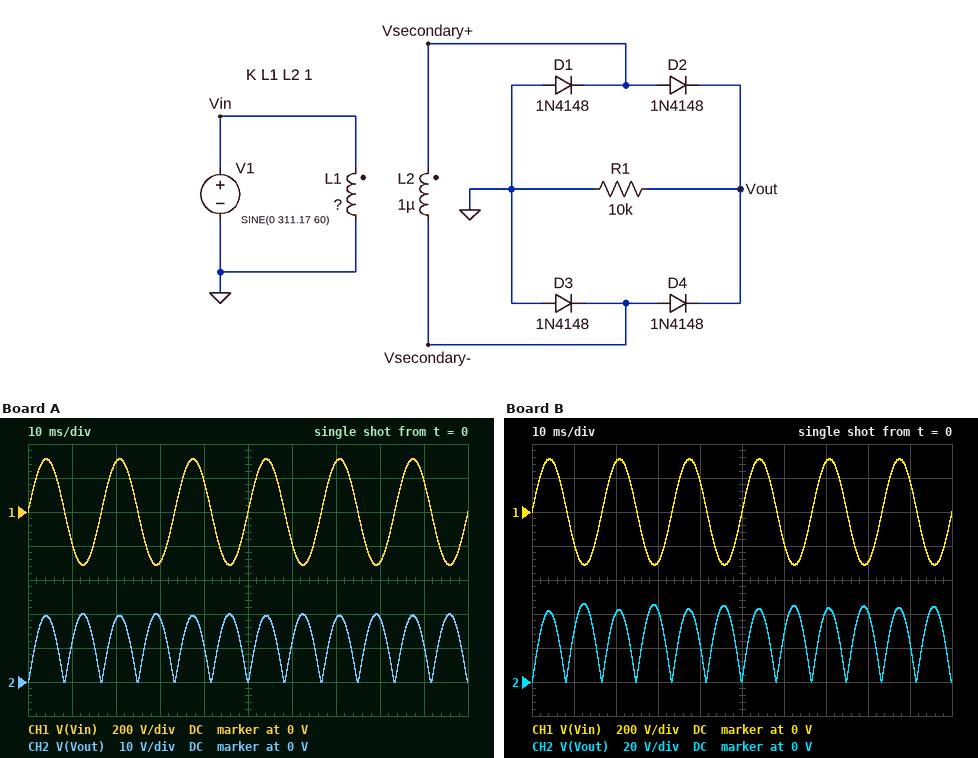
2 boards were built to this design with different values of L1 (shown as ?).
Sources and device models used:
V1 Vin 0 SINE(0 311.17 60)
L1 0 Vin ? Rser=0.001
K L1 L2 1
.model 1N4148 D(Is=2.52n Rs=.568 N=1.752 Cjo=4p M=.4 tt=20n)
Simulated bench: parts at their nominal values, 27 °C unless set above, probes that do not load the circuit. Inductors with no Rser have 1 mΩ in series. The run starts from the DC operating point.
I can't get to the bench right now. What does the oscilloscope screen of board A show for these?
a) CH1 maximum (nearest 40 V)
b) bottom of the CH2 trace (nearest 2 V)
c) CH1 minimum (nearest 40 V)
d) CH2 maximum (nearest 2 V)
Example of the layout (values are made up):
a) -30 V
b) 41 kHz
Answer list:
a) 320 V
b) 0 V
c) -320 V
d) 20 V
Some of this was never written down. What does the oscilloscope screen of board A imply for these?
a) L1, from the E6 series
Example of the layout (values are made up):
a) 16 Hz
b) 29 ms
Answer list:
a) 220 µH
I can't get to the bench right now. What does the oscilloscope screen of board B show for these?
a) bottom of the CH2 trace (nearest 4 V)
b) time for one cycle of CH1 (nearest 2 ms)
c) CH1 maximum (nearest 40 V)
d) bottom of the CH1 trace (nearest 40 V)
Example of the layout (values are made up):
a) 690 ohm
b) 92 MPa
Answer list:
a) 0 V
b) 16 ms
c) 320 V
d) -320 V
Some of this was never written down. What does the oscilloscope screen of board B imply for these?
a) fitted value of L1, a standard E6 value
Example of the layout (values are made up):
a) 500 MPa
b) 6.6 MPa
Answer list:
a) 47 µH
